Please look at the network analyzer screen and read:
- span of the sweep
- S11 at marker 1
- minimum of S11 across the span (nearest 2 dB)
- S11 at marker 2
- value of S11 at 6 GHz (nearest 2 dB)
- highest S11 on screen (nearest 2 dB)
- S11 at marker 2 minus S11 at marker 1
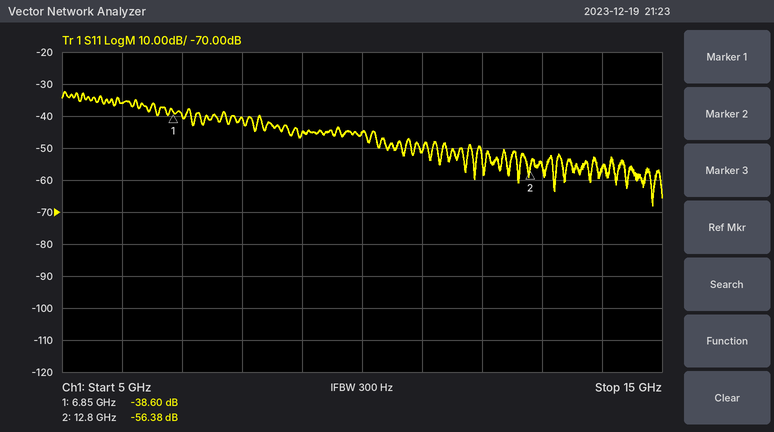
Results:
10 GHz
-38.60 dB
-68 dB
-56.38 dB
-36 dB
-32 dB
-17.78 dB
